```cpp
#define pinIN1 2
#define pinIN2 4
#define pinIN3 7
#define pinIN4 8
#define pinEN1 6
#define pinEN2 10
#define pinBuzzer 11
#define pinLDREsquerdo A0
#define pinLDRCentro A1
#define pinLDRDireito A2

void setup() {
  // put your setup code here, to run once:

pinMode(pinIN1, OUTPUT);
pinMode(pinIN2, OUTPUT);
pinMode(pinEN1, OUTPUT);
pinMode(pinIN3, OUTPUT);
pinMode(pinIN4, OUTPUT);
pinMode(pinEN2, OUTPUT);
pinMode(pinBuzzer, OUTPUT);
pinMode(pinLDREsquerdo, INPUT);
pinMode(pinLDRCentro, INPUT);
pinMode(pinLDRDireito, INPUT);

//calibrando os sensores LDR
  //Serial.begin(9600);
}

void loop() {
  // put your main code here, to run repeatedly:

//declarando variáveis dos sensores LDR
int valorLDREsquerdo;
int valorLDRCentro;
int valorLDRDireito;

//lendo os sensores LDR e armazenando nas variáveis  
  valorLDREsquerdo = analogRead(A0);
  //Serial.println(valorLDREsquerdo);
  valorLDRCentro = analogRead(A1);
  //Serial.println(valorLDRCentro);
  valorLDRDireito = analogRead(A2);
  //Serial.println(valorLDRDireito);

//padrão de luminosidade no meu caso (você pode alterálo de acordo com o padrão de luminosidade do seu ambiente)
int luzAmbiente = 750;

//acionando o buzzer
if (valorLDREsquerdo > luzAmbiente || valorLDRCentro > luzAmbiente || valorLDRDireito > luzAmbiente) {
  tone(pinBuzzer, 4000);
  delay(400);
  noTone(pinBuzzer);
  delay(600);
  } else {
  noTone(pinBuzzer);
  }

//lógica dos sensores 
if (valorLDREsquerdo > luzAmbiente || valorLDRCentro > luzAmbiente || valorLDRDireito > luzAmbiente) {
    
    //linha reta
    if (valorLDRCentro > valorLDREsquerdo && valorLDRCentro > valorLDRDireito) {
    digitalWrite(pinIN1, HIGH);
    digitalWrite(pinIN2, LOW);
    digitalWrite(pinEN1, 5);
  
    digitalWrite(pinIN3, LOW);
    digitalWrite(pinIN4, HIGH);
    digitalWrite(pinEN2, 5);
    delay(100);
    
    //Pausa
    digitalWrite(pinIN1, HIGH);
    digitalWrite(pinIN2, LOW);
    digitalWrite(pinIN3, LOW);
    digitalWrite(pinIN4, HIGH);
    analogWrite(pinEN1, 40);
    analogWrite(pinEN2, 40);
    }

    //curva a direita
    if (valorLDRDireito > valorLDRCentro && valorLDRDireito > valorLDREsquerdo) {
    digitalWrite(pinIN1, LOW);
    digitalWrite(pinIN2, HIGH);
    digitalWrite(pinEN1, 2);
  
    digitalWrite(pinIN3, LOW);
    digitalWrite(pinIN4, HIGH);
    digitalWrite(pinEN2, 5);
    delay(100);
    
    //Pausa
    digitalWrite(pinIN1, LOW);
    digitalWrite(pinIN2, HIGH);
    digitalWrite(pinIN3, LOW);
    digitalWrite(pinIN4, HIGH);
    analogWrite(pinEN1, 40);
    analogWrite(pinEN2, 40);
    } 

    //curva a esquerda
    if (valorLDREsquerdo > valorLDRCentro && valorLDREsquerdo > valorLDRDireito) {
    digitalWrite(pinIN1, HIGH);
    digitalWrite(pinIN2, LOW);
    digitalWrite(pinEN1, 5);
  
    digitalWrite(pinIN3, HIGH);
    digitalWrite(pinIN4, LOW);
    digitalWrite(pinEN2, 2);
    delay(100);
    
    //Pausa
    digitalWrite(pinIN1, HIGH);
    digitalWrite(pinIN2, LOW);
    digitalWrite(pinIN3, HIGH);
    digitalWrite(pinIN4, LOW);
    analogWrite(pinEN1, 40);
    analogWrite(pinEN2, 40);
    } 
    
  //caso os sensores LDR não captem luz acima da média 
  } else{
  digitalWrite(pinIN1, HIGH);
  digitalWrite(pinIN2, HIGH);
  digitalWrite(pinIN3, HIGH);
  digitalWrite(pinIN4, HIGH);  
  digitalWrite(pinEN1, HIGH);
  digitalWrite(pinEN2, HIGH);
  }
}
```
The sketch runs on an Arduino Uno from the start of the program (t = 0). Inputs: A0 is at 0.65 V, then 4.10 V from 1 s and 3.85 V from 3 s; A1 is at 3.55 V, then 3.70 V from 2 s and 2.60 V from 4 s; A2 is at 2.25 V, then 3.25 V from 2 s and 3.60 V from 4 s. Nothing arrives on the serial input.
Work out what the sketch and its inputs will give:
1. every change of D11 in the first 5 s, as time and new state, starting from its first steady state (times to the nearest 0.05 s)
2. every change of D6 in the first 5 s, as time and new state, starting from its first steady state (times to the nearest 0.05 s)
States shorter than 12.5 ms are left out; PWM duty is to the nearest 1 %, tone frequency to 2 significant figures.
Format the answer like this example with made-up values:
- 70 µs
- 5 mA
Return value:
- 0 s low; 1 s tone 4000 Hz; 1.4 s low; 2.1 s tone 4000 Hz; 2.5 s low; 3.2 s tone 4000 Hz; 3.6 s low; 4.3 s tone 4000 Hz; 4.7 s low
- 0 s high; 2.1 s PWM 16 %; 3.1 s high; 3.2 s PWM 16 %; 4.2 s high; 4.3 s PWM 16 %
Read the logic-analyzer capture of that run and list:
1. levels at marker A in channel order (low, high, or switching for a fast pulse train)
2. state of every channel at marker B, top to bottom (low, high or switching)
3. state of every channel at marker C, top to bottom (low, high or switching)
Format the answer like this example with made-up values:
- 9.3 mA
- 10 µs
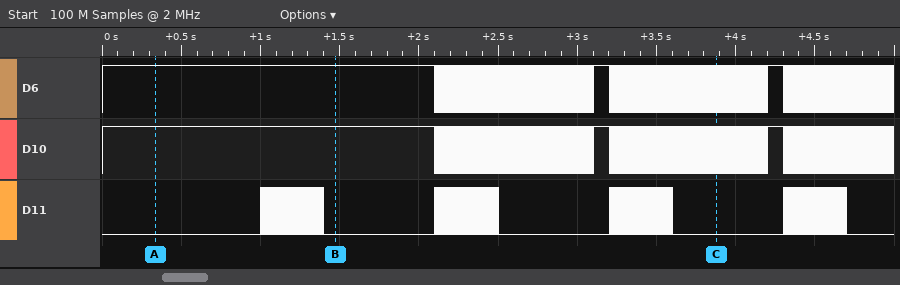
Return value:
- D6 high, D10 high, D11 low
- D6 high, D10 high, D11 low
- D6 switching, D10 switching, D11 low
